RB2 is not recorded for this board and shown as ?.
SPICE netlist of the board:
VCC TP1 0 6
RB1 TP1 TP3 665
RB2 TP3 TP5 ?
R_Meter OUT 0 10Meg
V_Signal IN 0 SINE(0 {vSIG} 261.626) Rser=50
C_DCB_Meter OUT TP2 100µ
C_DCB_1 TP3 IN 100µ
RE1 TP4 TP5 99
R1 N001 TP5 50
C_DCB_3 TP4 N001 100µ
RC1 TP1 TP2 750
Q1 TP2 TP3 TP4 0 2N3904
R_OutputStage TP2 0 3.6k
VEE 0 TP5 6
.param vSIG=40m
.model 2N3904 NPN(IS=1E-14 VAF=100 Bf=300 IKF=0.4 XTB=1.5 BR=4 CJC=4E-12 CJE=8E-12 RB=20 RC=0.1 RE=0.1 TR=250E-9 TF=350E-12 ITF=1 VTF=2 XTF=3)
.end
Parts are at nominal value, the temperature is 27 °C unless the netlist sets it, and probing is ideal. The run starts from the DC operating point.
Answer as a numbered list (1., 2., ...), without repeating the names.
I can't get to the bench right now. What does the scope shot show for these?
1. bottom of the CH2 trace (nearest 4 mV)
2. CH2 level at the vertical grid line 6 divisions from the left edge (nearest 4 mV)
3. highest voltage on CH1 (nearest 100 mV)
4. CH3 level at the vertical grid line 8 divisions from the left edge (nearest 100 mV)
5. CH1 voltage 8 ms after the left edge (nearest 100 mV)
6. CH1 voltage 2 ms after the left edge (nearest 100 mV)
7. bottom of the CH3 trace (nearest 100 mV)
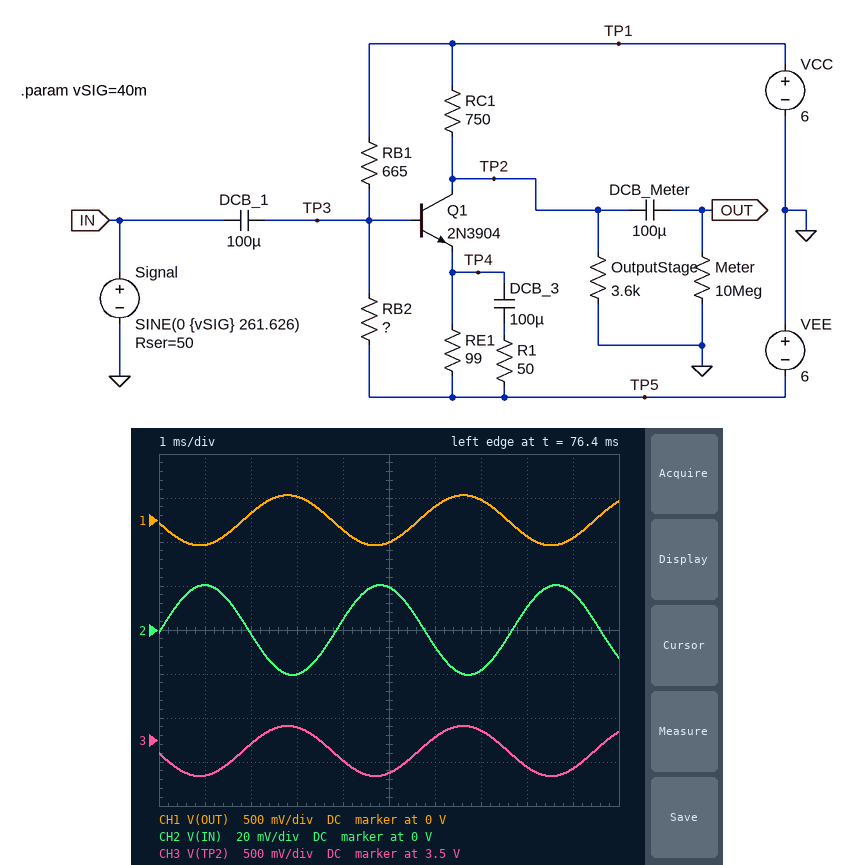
1. -20 mV
2. -8 mV
3. 300 mV
4. 3.2 V
5. -200 mV
6. 100 mV
7. 3.1 V
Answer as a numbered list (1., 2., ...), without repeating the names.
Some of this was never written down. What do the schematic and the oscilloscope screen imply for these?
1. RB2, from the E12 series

1. 56 Ω
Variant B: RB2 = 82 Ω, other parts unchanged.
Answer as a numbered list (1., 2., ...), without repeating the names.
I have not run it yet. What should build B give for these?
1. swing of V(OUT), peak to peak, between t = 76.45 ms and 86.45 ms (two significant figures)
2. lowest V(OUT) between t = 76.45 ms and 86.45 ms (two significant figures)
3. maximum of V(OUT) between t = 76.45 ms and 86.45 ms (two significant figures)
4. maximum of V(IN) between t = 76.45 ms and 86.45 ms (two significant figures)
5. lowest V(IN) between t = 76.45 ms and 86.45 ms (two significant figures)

1. 770 mV
2. -390 mV
3. 380 mV
4. 24 mV
5. -24 mV
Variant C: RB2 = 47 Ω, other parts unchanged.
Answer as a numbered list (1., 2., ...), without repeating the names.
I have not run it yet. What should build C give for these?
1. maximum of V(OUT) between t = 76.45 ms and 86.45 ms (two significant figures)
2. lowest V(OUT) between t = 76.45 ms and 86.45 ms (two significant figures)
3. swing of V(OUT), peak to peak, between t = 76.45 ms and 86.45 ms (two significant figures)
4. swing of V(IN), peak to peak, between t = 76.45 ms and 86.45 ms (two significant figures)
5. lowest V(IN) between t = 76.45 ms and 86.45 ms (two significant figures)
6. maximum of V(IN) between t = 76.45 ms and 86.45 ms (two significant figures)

1. 210 mV
2. -220 mV
3. 430 mV
4. 38 mV
5. -19 mV
6. 19 mV
